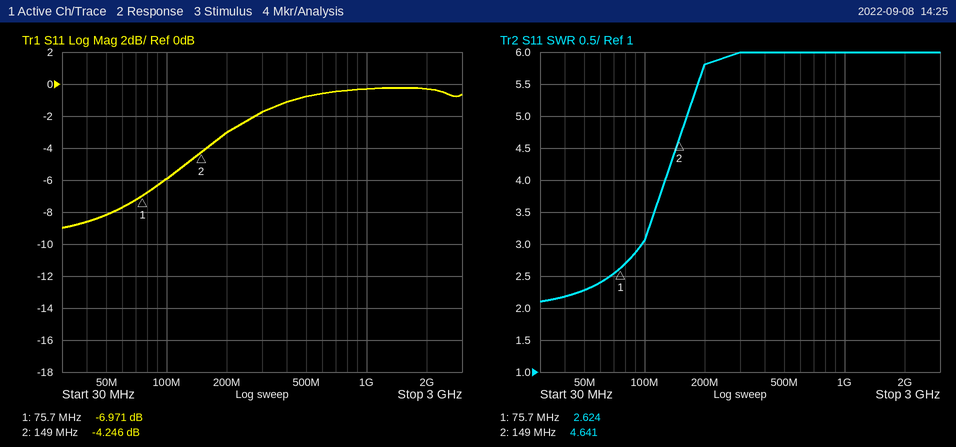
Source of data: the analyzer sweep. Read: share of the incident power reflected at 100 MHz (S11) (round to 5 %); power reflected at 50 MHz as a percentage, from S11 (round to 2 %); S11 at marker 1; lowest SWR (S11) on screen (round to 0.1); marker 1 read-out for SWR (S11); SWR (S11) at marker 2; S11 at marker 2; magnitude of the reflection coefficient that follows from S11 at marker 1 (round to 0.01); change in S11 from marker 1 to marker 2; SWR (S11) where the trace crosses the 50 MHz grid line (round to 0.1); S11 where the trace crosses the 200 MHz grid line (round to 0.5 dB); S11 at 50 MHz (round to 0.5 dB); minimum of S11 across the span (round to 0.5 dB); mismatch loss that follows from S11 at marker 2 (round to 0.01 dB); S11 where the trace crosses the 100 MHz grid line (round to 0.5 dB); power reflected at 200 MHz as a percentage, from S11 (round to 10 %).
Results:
25 %
16 %
-6.971 dB
2.1
2.624
4.641
-4.246 dB
0.45
2.725 dB
2.3
-3.0 dB
-8.0 dB
-9.0 dB
2.05 dB
-6.0 dB
50 %
